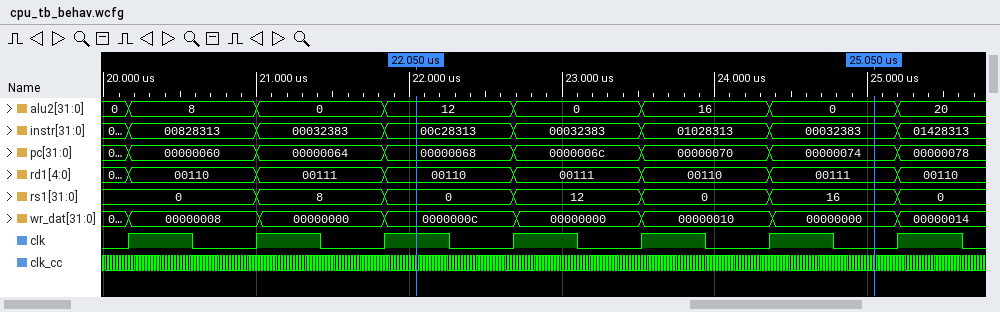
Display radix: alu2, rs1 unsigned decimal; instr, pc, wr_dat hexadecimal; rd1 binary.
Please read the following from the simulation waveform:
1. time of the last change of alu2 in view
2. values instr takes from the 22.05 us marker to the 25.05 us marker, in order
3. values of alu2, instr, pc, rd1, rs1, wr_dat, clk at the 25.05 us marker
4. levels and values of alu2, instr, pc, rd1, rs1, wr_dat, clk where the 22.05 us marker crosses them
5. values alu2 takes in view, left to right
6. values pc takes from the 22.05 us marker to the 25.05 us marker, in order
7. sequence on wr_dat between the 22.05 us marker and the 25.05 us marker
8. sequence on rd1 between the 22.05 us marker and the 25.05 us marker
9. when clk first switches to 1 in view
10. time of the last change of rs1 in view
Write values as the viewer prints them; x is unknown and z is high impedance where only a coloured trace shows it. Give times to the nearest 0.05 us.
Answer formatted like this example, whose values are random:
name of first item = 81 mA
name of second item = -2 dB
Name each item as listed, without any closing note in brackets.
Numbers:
time of the last change of alu2 in view = 25.2 us
values instr takes from the 22.05 us marker to the 25.05 us marker, in order = 00c28313, 00032383, 01028313, 00032383
values of alu2, instr, pc, rd1, rs1, wr_dat, clk at the 25.05 us marker = alu2=0, instr=00032383, pc=00000074, rd1=00111, rs1=16, wr_dat=00000000, clk=0
levels and values of alu2, instr, pc, rd1, rs1, wr_dat, clk where the 22.05 us marker crosses them = alu2=12, instr=00c28313, pc=00000068, rd1=00110, rs1=0, wr_dat=0000000c, clk=1
values alu2 takes in view, left to right = 0, 8, 0, 12, 0, 16, 0, 20
values pc takes from the 22.05 us marker to the 25.05 us marker, in order = 00000068, 0000006c, 00000070, 00000074
sequence on wr_dat between the 22.05 us marker and the 25.05 us marker = 0000000c, 00000000, 00000010, 00000000
sequence on rd1 between the 22.05 us marker and the 25.05 us marker = 00110, 00111, 00110, 00111
when clk first switches to 1 in view = 20.15 us
time of the last change of rs1 in view = 25.2 us
